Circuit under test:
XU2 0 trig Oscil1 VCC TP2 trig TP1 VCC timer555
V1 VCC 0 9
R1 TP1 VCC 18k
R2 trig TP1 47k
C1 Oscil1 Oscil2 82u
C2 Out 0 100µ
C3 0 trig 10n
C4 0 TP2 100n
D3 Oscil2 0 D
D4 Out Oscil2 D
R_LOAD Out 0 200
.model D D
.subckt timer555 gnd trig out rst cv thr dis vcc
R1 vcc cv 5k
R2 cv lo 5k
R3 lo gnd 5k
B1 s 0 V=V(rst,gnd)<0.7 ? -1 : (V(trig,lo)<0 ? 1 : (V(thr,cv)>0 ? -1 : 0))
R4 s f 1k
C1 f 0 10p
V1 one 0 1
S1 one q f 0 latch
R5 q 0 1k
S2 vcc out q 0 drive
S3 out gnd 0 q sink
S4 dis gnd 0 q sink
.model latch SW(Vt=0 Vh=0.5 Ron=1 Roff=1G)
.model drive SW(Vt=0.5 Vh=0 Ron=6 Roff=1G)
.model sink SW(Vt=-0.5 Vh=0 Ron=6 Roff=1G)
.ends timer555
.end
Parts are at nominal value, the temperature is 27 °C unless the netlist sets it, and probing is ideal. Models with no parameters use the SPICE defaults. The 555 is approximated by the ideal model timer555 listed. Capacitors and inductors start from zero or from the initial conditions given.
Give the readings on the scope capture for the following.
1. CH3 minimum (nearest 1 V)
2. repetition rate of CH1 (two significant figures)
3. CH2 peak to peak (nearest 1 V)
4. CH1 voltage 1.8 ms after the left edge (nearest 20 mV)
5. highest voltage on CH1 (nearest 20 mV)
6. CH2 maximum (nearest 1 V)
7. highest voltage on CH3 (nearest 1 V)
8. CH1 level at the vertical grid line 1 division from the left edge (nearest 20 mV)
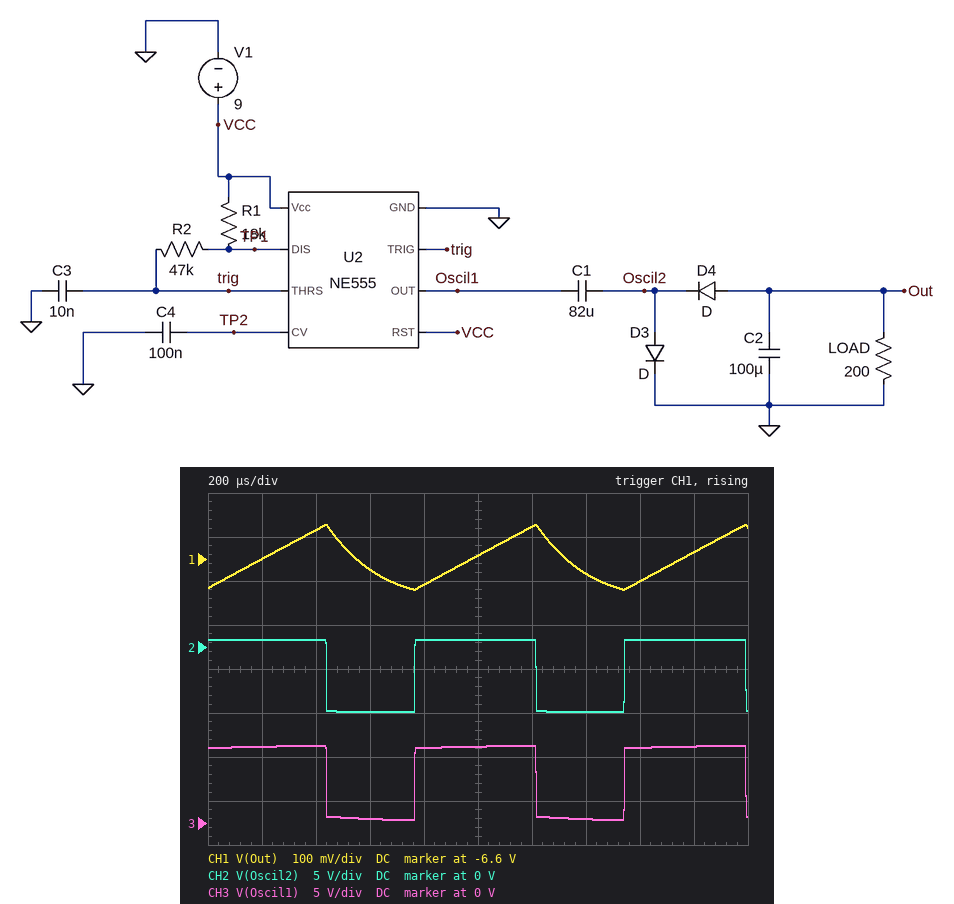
0 V
1.3 kHz
8 V
-6.58 V
-6.52 V
1 V
9 V
-6.60 V
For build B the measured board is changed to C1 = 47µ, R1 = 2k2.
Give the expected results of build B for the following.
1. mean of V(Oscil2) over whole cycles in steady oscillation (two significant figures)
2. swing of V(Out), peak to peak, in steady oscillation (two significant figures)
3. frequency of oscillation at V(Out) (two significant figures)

-3.2 V
110 mV
1.5 kHz
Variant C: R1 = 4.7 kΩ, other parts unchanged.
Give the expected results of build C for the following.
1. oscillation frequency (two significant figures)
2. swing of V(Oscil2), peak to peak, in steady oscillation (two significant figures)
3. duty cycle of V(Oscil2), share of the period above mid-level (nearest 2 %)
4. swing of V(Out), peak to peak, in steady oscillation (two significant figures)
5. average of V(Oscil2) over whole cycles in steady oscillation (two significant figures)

1.5 kHz
8.2 V
52 %
120 mV
-3.1 V
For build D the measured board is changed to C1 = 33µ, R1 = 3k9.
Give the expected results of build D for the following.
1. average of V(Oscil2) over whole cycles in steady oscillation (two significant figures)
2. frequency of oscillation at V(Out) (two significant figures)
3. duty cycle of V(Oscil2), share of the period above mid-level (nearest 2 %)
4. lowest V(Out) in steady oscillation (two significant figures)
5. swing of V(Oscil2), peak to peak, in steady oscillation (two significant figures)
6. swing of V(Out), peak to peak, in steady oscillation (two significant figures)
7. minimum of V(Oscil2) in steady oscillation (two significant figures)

-3.1 V
1.5 kHz
52 %
-6.5 V
8.1 V
120 mV
-7.3 V
